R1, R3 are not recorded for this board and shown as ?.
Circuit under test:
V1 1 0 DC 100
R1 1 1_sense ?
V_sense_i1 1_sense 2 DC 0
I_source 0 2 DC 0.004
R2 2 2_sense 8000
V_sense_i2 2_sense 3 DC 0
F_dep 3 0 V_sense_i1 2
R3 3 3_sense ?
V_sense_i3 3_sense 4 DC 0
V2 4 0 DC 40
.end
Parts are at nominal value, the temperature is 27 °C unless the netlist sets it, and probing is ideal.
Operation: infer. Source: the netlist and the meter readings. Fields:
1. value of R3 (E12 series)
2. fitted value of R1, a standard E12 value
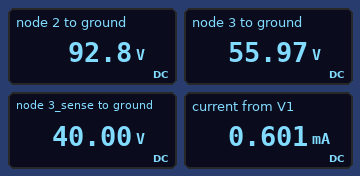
4.7 kΩ
12 kΩ
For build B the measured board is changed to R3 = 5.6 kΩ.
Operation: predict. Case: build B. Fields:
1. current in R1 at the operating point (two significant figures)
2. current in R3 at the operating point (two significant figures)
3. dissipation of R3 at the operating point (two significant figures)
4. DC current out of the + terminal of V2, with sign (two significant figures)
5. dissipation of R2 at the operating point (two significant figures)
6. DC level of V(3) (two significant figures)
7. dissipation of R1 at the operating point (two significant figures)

390 µA
3.6 mA
73 mW
-3.6 mA
150 mW
60 V
1.8 mW
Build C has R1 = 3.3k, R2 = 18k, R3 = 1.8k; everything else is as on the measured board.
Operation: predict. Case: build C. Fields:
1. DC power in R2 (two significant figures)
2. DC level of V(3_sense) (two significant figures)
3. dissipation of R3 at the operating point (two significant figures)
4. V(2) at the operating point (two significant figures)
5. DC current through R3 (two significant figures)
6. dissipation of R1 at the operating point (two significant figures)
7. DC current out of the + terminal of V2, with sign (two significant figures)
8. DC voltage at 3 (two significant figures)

160 mW
40 V
45 mW
100 V
5.0 mA
3.2 mW
-5.0 mA
49 V
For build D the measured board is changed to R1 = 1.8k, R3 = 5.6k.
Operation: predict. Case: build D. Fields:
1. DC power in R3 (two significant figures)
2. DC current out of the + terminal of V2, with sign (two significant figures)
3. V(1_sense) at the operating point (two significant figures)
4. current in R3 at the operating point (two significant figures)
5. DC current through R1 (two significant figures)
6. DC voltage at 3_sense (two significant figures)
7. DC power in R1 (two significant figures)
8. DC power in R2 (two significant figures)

40 mW
-2.7 mA
98 V
2.7 mA
1.3 mA
40 V
3.2 mW
230 mW
